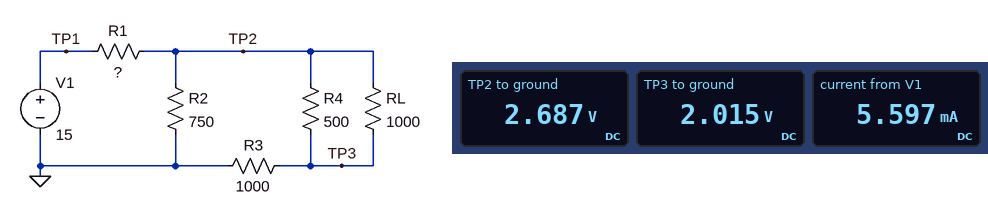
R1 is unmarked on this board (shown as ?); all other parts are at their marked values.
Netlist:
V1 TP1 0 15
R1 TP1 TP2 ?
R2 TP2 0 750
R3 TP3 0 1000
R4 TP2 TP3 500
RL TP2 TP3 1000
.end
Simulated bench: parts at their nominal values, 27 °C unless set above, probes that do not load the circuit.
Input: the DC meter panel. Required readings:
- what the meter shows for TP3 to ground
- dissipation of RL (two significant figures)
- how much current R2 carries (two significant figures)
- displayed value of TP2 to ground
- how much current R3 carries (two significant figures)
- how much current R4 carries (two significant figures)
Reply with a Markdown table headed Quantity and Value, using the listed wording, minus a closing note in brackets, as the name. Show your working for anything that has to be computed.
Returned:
| Quantity | Value |
|---|---|
| what the meter shows for TP3 to ground | 2.015 V |
| dissipation of RL | (2.687 V - 2.015 V)^2 / 1 kΩ = 450 µW |
| how much current R2 carries | (2.687 V) / 750 Ω = 3.6 mA |
| displayed value of TP2 to ground | 2.687 V |
| how much current R3 carries | (2.015 V) / 1 kΩ = 2.0 mA |
| how much current R4 carries | (2.687 V - 2.015 V) / 500 Ω = 1.3 mA |
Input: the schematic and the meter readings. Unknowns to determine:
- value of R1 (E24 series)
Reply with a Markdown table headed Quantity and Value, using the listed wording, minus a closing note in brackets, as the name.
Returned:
| Quantity | Value |
|---|---|
| value of R1 | 2.2 kΩ |
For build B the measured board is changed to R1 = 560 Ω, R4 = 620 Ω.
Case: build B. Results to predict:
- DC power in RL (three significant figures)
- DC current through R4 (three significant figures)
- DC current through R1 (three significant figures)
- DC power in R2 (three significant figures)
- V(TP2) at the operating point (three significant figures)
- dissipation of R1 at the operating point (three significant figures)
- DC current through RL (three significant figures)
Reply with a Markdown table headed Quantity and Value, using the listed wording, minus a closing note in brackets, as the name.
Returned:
| Quantity | Value |
|---|---|
| DC power in RL | 3.72 mW |
| DC current through R4 | 3.11 mA |
| DC current through R1 | 14.3 mA |
| DC power in R2 | 64.8 mW |
| V(TP2) at the operating point | 6.97 V |
| dissipation of R1 at the operating point | 115 mW |
| DC current through RL | 1.93 mA |
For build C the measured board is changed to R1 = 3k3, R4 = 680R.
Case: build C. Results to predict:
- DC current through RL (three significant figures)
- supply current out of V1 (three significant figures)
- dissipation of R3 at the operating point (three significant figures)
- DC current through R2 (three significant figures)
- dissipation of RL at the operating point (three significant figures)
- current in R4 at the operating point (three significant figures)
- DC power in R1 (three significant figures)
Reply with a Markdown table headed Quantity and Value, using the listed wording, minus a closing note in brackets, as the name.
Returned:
| Quantity | Value |
|---|---|
| DC current through RL | 558 µA |
| supply current out of V1 | 3.96 mA |
| dissipation of R3 at the operating point | 1.90 mW |
| DC current through R2 | 2.58 mA |
| dissipation of RL at the operating point | 311 µW |
| current in R4 at the operating point | 820 µA |
| DC power in R1 | 51.7 mW |
